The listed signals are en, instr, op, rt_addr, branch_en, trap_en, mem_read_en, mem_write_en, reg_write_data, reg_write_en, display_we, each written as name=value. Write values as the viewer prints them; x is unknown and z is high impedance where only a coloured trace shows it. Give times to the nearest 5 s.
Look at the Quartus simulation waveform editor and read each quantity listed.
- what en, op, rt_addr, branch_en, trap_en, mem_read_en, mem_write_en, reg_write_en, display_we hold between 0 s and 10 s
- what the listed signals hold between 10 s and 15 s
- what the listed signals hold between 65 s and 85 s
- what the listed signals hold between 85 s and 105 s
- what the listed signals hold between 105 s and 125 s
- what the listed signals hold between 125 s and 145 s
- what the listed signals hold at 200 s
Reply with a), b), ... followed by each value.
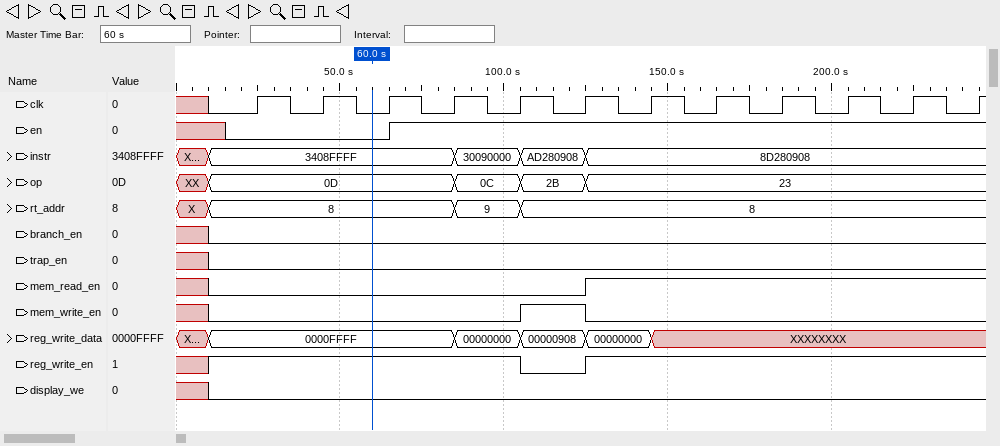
a) en=x, op=XX, rt_addr=X, branch_en=x, trap_en=x, mem_read_en=x, mem_write_en=x, reg_write_en=x, display_we=x
b) en=x, instr=3408FFFF, op=0D, rt_addr=8, branch_en=0, trap_en=0, mem_read_en=0, mem_write_en=0, reg_write_data=0000FFFF, reg_write_en=1, display_we=0
c) en=1, instr=3408FFFF, op=0D, rt_addr=8, branch_en=0, trap_en=0, mem_read_en=0, mem_write_en=0, reg_write_data=0000FFFF, reg_write_en=1, display_we=0
d) en=1, instr=30090000, op=0C, rt_addr=9, branch_en=0, trap_en=0, mem_read_en=0, mem_write_en=0, reg_write_data=00000000, reg_write_en=1, display_we=0
e) en=1, instr=AD280908, op=2B, rt_addr=8, branch_en=0, trap_en=0, mem_read_en=0, mem_write_en=1, reg_write_data=00000908, reg_write_en=0, display_we=0
f) en=1, instr=8D280908, op=23, rt_addr=8, branch_en=0, trap_en=0, mem_read_en=1, mem_write_en=0, reg_write_data=00000000, reg_write_en=1, display_we=0
g) en=1, instr=8D280908, op=23, rt_addr=8, branch_en=0, trap_en=0, mem_read_en=1, mem_write_en=0, reg_write_data=XXXXXXXX, reg_write_en=1, display_we=0
